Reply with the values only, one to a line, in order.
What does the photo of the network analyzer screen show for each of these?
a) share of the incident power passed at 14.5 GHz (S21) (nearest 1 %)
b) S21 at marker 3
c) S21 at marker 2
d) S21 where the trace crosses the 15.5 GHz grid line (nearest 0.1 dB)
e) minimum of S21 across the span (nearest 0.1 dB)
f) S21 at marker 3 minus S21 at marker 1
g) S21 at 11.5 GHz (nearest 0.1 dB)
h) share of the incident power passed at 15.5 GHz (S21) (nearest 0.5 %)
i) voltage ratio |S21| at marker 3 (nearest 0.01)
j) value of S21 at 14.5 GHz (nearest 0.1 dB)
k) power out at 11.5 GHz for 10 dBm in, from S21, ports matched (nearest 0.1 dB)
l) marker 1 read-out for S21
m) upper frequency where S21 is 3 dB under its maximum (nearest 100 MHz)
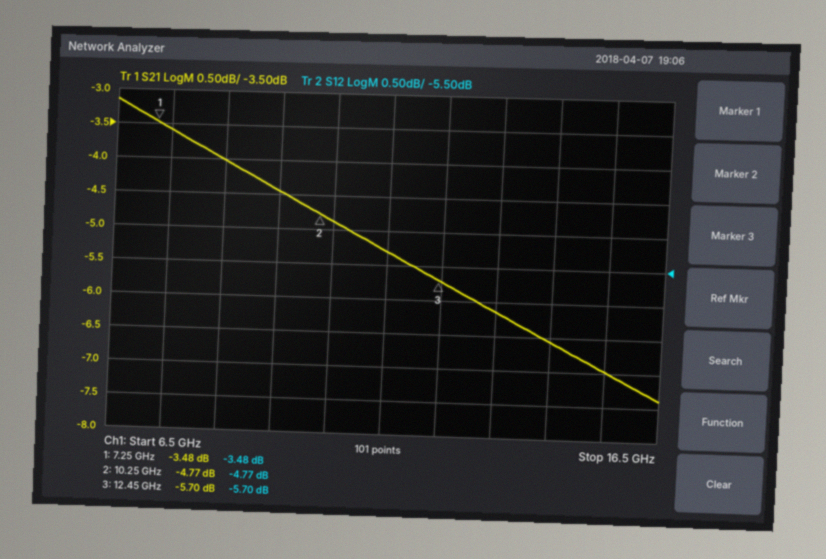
22 %
-5.70 dB
-4.77 dB
-7.0 dB
-7.4 dB
-2.22 dB
-5.3 dB
20.0 %
0.52
-6.6 dB
4.7 dBm
-3.48 dB
13.5 GHz
